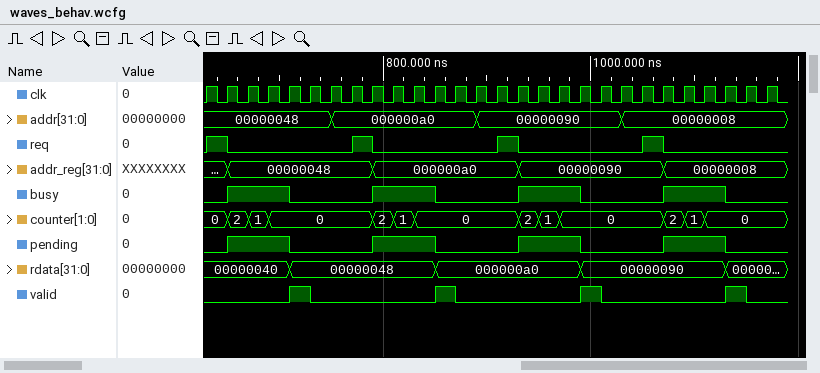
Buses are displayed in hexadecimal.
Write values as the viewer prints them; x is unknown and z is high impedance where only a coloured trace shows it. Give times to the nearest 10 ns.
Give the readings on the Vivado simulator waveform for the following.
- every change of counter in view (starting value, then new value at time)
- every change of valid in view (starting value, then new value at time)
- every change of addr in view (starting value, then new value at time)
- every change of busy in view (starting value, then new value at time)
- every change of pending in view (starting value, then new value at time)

0, 2 at 650 ns, 1 at 670 ns, 0 at 690 ns, 2 at 790 ns, 1 at 810 ns, 0 at 830 ns, 2 at 930 ns, 1 at 950 ns, 0 at 970 ns, 2 at 1070 ns, 1 at 1090 ns, 0 at 1110 ns
0, 1 at 710 ns, 0 at 730 ns, 1 at 850 ns, 0 at 870 ns, 1 at 990 ns, 0 at 1010 ns, 1 at 1130 ns, 0 at 1150 ns
00000048, 000000a0 at 750 ns, 00000090 at 890 ns, 00000008 at 1030 ns
0, 1 at 650 ns, 0 at 710 ns, 1 at 790 ns, 0 at 850 ns, 1 at 930 ns, 0 at 990 ns, 1 at 1070 ns, 0 at 1130 ns
0, 1 at 650 ns, 0 at 710 ns, 1 at 790 ns, 0 at 850 ns, 1 at 930 ns, 0 at 990 ns, 1 at 1070 ns, 0 at 1130 ns
